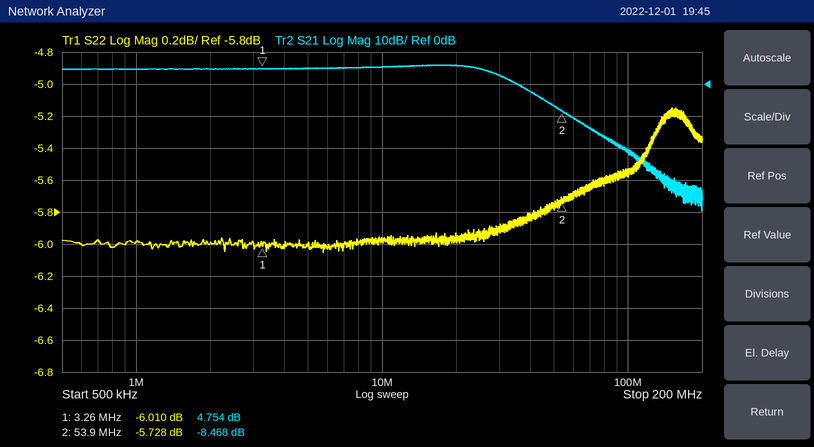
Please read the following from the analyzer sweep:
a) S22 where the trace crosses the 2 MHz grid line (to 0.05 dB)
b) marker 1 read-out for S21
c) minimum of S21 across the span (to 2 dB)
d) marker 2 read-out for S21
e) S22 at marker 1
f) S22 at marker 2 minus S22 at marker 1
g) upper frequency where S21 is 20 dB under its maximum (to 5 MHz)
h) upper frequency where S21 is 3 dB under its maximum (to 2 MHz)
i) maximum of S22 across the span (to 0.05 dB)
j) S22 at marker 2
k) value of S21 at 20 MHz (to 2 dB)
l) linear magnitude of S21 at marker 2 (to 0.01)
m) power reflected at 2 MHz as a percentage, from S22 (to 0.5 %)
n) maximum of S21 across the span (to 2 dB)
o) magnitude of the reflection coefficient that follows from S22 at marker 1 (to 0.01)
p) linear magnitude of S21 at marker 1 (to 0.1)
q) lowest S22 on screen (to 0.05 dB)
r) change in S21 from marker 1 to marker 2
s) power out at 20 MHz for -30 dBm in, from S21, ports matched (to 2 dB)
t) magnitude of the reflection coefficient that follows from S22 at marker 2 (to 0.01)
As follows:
-6.00 dB
4.754 dB
-40 dB
-8.468 dB
-6.010 dB
0.282 dB
70 MHz
30 MHz
-5.15 dB
-5.728 dB
6 dB
0.38
25.0 %
6 dB
0.50
1.7
-6.05 dB
-13.222 dB
-24 dBm
0.52
